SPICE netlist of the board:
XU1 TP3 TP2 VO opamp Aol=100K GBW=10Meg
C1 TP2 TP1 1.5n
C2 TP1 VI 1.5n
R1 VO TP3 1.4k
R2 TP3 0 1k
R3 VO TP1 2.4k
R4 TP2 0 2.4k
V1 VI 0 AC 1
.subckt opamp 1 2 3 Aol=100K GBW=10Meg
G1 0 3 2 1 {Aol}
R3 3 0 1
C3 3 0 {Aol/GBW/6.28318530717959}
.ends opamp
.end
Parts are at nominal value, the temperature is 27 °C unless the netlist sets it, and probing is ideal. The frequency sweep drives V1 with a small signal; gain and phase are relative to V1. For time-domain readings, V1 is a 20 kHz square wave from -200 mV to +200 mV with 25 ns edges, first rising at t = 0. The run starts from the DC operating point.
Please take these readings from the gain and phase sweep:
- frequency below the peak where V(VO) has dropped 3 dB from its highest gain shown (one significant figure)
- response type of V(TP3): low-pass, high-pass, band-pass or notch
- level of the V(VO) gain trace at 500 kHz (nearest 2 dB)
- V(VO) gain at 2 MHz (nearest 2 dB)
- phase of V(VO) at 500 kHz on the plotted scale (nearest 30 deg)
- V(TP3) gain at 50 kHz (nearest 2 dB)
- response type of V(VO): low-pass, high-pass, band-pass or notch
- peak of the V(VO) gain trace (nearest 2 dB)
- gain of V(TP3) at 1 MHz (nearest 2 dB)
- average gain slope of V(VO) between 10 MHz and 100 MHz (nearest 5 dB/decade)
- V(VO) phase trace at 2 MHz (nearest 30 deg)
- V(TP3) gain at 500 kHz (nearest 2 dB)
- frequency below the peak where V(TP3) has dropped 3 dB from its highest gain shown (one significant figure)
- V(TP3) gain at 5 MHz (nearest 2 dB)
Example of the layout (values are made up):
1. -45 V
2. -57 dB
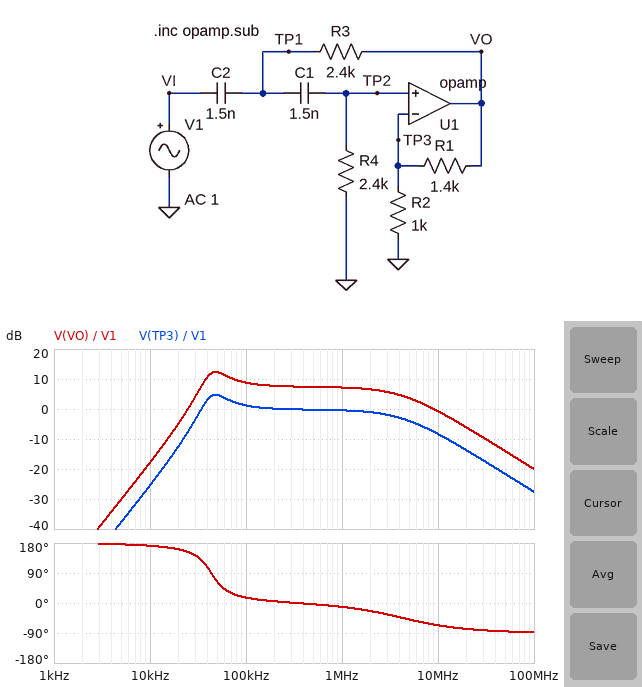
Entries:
1. 40 kHz
2. band-pass
3. 8 dB
4. 6 dB
5. 0 deg
6. 4 dB
7. band-pass
8. 12 dB
9. 0 dB
10. -20 dB/decade
11. -30 deg
12. 0 dB
13. 40 kHz
14. -4 dB
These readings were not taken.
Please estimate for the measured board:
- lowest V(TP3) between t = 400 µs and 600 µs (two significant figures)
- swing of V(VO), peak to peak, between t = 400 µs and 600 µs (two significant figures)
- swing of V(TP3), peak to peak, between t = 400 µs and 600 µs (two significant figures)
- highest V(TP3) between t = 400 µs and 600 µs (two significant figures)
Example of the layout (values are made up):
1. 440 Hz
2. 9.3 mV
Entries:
1. -340 mV
2. 1.6 V
3. 680 mV
4. 340 mV
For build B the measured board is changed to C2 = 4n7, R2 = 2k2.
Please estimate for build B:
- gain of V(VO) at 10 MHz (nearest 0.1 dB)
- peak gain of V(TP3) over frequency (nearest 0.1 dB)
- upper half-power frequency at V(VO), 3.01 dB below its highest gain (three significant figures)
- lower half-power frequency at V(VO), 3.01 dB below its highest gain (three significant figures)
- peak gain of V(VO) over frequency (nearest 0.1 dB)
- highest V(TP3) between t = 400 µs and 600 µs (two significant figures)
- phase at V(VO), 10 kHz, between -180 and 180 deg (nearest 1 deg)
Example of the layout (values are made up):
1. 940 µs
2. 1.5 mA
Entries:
1. -1.4 dB
2. -0.1 dB
3. 6.20 MHz
4. 37.6 kHz
5. 4.2 dB
6. 410 mV
7. 137 deg
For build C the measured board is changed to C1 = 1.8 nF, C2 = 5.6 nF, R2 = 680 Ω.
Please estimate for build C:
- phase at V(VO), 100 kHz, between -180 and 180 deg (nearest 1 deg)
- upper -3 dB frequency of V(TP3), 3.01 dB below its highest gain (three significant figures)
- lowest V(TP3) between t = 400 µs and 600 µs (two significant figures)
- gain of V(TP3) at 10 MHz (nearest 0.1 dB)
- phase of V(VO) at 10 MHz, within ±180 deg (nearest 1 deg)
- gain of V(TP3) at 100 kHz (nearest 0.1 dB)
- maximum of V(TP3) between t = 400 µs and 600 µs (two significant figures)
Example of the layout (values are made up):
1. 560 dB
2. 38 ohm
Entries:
1. 12 deg
2. 2.92 MHz
3. -470 mV
4. -10.2 dB
5. -72 deg
6. 0 dB
7. 470 mV
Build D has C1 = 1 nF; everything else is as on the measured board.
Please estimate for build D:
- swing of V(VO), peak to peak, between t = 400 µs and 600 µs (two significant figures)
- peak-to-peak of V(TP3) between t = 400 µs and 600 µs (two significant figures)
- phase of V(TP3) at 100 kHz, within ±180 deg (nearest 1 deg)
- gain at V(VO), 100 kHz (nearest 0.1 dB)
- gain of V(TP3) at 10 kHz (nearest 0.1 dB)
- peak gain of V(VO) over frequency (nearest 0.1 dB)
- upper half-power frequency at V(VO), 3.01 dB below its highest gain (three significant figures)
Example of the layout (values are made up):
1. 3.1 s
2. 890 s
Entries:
1. 1.8 V
2. 750 mV
3. 32 deg
4. 8.7 dB
5. -29.2 dB
6. 9.4 dB
7. 2.20 MHz
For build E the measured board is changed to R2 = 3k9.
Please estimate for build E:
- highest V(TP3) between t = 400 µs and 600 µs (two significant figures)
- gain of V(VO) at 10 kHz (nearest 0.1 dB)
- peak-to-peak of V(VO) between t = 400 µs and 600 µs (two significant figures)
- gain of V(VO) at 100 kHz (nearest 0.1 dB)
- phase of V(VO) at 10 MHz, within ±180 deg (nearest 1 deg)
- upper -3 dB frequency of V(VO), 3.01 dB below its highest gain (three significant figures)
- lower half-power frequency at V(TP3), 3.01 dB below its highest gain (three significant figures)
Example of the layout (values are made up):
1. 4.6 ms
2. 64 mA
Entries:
1. 380 mV
2. -23.3 dB
3. 1.0 V
4. 1.9 dB
5. -53 deg
6. 7.49 MHz
7. 51.6 kHz
